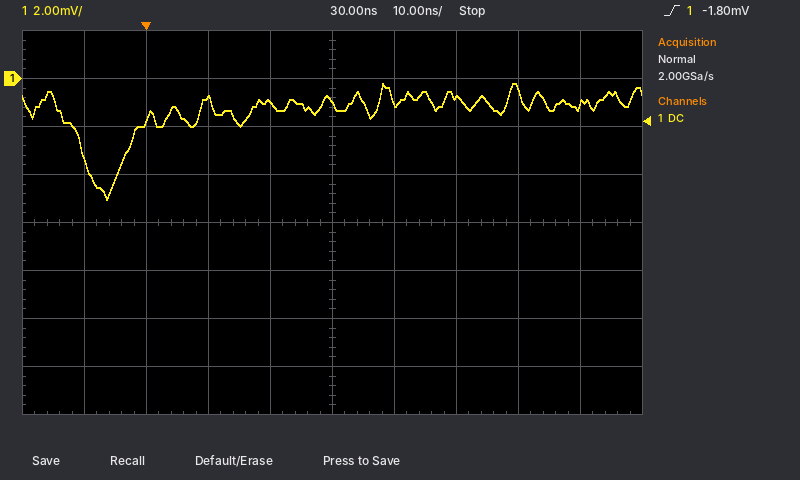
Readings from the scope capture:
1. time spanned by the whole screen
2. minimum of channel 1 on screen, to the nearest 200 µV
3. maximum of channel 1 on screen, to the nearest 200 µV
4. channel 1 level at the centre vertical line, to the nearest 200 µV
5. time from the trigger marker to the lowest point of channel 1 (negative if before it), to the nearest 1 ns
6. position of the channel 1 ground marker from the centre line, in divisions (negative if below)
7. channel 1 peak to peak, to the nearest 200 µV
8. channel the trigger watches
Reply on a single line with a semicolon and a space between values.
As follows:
100 ns; -5.0 mV; -200 µV; -1.0 mV; -6 ns; +3.0 div; 4.8 mV; channel 1
